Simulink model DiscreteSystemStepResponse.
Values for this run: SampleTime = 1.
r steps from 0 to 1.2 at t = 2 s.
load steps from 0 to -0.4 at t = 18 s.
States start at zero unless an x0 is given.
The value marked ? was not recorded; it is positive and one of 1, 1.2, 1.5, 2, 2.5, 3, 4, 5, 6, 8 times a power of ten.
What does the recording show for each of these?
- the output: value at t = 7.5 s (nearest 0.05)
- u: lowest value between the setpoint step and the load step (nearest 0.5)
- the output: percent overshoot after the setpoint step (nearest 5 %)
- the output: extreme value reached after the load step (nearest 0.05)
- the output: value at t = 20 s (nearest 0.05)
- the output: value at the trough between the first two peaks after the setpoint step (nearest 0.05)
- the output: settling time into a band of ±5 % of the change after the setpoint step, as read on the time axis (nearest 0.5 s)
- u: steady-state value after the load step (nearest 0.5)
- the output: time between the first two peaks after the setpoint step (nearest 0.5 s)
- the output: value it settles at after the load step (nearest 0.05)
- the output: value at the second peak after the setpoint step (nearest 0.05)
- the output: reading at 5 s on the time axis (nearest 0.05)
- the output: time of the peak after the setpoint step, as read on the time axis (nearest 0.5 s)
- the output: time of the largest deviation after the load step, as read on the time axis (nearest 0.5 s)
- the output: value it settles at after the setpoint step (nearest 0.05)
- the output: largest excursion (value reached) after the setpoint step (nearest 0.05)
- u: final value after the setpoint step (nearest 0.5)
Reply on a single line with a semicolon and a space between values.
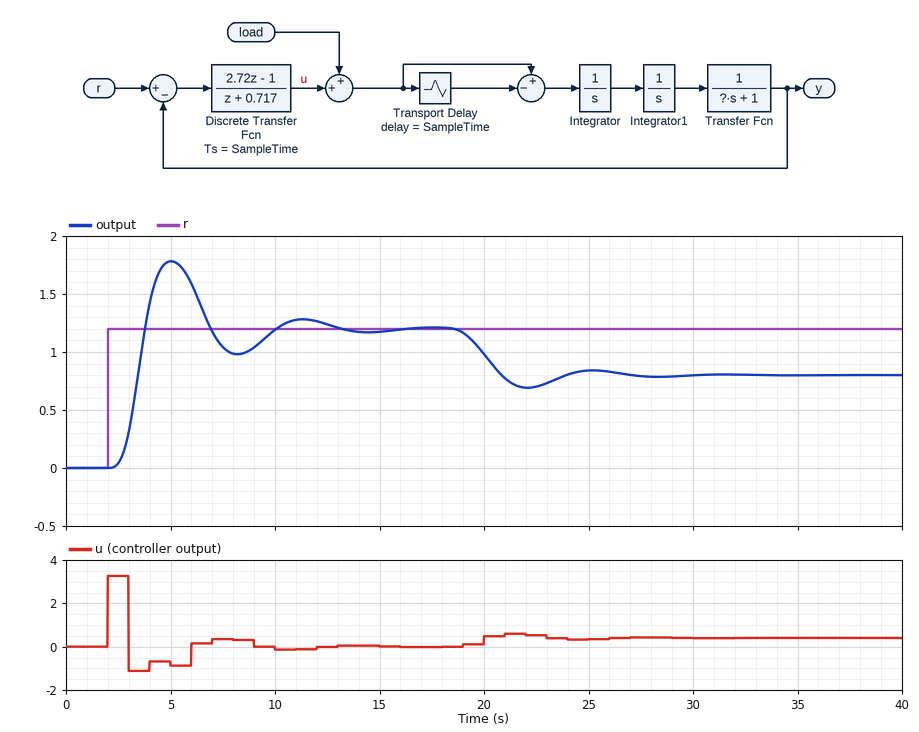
1.05; -1.0; 50 %; 0.70; 1.00; 1.00; 12.0 s; 0.5; 6.5 s; 0.80; 1.30; 1.80; 5.0 s; 22.0 s; 1.20; 1.80; 0.0
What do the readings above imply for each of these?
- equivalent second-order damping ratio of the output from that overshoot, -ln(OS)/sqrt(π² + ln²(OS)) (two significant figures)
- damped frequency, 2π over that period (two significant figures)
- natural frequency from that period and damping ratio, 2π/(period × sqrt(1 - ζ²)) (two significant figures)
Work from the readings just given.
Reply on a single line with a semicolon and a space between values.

0.22; 0.97 rad/s; 0.99 rad/s
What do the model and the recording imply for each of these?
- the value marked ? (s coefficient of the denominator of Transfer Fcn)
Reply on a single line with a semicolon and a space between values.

1.5
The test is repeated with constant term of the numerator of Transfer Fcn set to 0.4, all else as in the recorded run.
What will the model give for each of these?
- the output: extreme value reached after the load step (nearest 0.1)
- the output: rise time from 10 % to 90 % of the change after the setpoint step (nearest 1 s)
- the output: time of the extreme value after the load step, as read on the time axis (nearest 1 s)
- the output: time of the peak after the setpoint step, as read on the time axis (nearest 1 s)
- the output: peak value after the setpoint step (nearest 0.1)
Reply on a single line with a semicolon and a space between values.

0.8; 3 s; 26 s; 8 s; 1.3
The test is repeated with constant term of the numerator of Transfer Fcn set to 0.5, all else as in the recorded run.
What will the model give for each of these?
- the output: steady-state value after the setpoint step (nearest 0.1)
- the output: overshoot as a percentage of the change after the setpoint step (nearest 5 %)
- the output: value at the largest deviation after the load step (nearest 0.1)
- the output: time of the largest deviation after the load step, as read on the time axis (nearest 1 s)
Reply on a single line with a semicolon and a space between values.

1.2; 10 %; 0.8; 25 s
